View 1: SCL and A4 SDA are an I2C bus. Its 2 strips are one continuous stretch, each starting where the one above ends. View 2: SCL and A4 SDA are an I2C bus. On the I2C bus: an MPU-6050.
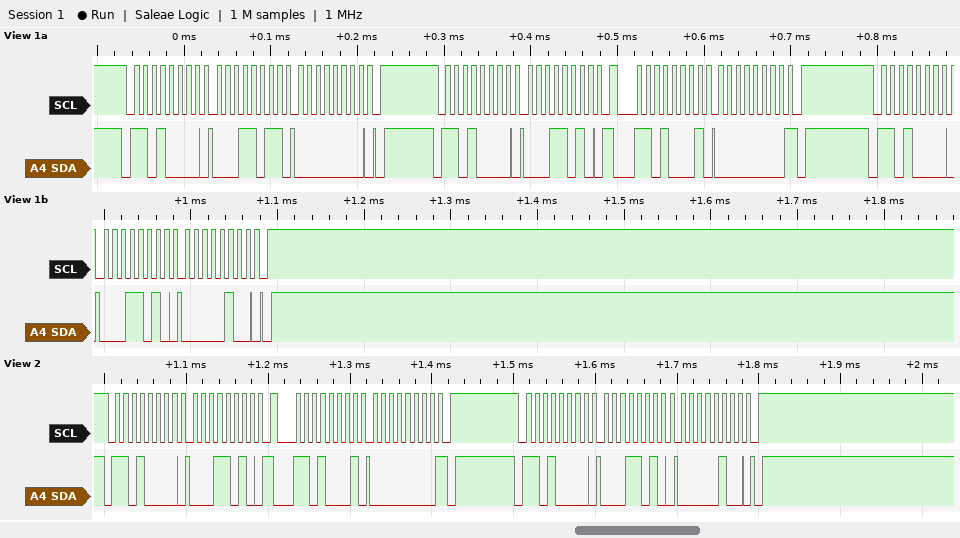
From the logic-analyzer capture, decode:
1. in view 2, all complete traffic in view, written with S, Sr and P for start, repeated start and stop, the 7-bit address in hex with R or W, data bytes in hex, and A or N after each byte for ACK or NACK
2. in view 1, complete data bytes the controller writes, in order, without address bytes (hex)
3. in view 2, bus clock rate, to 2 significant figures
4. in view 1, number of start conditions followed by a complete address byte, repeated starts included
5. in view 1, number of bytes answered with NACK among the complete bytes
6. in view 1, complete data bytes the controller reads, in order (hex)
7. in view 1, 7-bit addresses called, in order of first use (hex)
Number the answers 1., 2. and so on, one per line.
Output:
1. S 68W A 1A A Sr 68R A 00 N P S 68W A 1A A 04 A P
2. 1B 00 1A 1A 04
3. 100 kHz
4. 4
5. 1
6. 00
7. 0x68
